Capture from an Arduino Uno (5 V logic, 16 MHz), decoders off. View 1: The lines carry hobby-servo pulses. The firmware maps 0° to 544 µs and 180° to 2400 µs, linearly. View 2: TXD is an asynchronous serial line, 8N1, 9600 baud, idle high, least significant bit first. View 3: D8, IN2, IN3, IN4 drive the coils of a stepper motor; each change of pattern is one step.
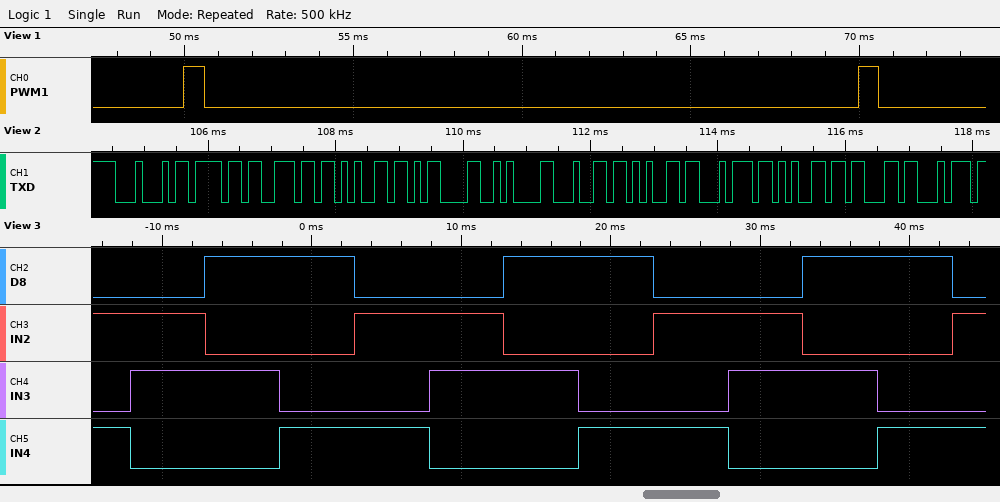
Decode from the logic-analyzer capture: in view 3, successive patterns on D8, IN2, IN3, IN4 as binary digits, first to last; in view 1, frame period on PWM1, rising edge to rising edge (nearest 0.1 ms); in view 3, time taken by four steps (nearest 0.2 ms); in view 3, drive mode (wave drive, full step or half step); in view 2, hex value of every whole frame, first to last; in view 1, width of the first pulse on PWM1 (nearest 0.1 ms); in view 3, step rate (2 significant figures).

0101 0110 1010 1001 0101 0110 1010 1001 0101 0110 1010 1001 0101
20.0 ms
20.0 ms
full step
44 6F 6E 65 0D 0A 64 65 74 65 63 74
0.6 ms
200 steps/s
